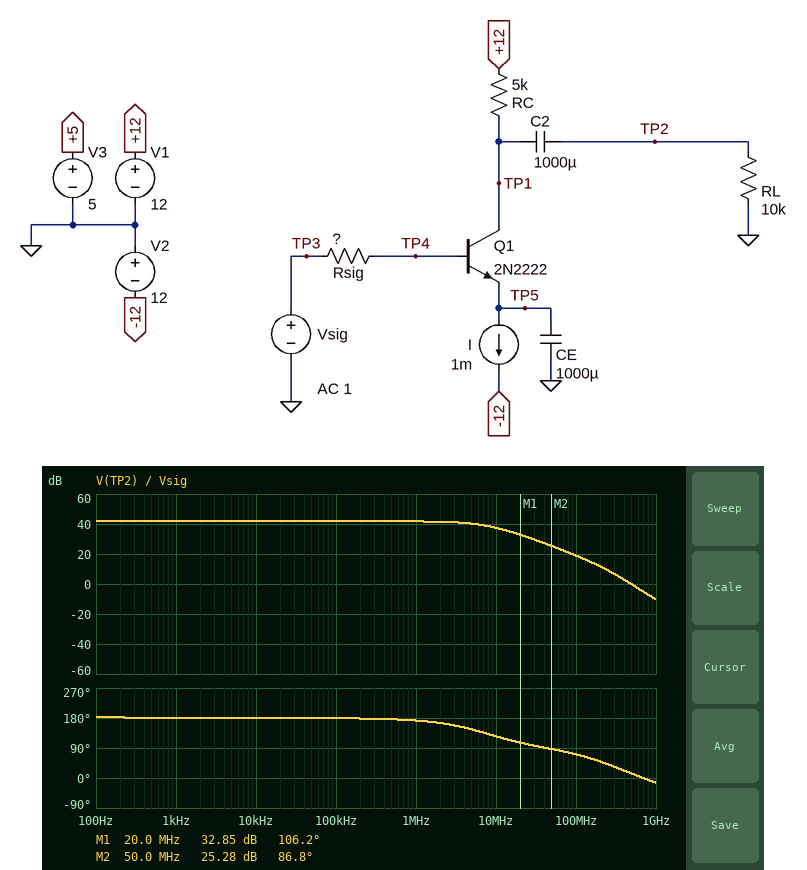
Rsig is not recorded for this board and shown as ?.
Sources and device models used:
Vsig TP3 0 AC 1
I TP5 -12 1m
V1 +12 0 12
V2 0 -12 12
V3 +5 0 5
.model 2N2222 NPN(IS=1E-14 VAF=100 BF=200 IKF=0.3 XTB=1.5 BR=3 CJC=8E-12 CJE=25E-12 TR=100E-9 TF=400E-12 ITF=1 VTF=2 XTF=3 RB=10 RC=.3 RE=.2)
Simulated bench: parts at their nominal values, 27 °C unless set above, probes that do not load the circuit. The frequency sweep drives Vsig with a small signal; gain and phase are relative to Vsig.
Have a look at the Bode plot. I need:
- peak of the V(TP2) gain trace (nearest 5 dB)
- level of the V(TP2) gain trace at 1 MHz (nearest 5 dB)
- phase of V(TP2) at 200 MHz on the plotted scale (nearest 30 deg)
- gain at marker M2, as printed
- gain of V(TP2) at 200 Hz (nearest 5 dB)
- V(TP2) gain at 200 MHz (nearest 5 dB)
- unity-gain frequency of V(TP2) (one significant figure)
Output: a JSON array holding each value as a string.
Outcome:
["40 dB", "40 dB", "60 deg", "25.28 dB", "40 dB", "10 dB", "500 MHz"]
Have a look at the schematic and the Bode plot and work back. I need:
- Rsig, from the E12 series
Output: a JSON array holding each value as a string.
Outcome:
["8.2 Ω"]
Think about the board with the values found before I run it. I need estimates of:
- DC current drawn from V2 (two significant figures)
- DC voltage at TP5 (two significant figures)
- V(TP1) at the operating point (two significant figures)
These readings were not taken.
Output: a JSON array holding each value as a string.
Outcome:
["1.0 mA", "-650 mV", "7.0 V"]
